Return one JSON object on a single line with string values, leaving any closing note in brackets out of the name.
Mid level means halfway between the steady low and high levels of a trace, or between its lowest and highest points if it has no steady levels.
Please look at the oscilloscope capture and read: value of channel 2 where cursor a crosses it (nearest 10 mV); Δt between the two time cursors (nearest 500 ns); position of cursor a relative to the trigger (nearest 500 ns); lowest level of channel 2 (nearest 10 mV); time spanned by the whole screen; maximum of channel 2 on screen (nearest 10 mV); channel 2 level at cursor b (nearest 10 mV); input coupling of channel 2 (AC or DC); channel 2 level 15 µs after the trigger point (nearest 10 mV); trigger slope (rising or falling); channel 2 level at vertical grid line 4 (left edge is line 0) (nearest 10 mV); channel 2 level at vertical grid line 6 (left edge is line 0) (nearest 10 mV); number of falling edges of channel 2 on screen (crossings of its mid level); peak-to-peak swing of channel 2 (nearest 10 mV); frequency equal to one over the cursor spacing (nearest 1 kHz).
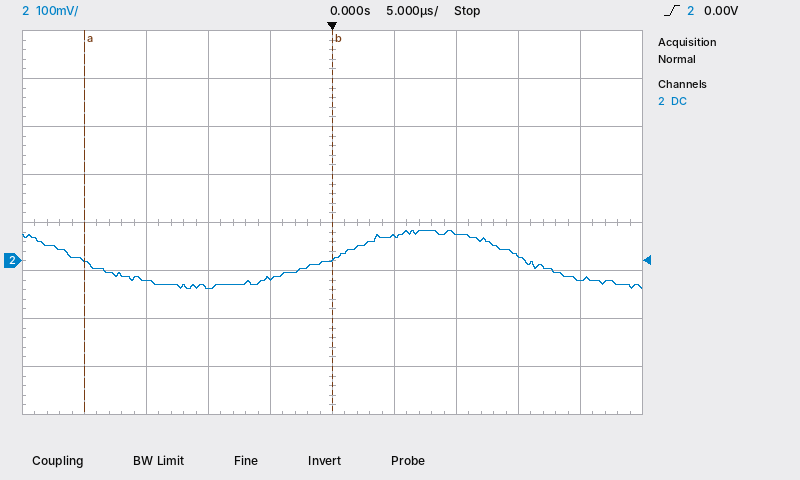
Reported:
{"value of channel 2 where cursor a crosses it": "0 mV", "Δt between the two time cursors": "20.0 µs", "position of cursor a relative to the trigger": "-20.0 µs", "lowest level of channel 2": "-60 mV", "time spanned by the whole screen": "50 µs", "maximum of channel 2 on screen": "60 mV", "channel 2 level at cursor b": "0 mV", "input coupling of channel 2": "DC", "channel 2 level 15 µs after the trigger point": "10 mV", "trigger slope": "rising", "channel 2 level at vertical grid line 4 (left edge is line 0)": "-40 mV", "channel 2 level at vertical grid line 6 (left edge is line 0)": "50 mV", "number of falling edges of channel 2 on screen": "2", "peak-to-peak swing of channel 2": "120 mV", "frequency equal to one over the cursor spacing": "50 kHz"}
